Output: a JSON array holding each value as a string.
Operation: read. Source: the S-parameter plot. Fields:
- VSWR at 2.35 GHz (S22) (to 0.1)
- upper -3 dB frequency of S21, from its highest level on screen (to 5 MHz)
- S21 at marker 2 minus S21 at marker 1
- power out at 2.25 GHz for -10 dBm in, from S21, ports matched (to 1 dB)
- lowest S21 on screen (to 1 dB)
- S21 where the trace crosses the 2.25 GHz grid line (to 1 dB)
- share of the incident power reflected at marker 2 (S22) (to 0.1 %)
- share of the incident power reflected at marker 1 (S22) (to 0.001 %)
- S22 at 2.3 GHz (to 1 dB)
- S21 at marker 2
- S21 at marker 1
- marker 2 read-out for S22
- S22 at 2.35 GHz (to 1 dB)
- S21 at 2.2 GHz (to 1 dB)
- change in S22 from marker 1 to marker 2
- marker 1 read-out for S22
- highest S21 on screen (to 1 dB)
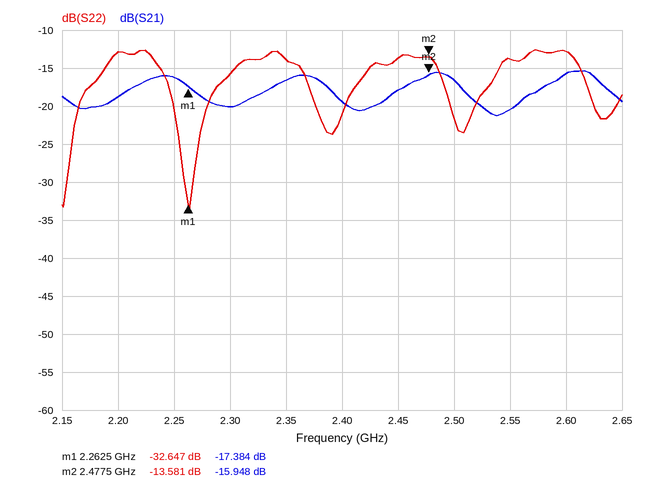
["1.5", "2.640 GHz", "1.436 dB", "-26 dBm", "-21 dB", "-16 dB", "4.4 %", "0.054 %", "-16 dB", "-15.948 dB", "-17.384 dB", "-13.581 dB", "-14 dB", "-19 dB", "19.066 dB", "-32.647 dB", "-15 dB"]
